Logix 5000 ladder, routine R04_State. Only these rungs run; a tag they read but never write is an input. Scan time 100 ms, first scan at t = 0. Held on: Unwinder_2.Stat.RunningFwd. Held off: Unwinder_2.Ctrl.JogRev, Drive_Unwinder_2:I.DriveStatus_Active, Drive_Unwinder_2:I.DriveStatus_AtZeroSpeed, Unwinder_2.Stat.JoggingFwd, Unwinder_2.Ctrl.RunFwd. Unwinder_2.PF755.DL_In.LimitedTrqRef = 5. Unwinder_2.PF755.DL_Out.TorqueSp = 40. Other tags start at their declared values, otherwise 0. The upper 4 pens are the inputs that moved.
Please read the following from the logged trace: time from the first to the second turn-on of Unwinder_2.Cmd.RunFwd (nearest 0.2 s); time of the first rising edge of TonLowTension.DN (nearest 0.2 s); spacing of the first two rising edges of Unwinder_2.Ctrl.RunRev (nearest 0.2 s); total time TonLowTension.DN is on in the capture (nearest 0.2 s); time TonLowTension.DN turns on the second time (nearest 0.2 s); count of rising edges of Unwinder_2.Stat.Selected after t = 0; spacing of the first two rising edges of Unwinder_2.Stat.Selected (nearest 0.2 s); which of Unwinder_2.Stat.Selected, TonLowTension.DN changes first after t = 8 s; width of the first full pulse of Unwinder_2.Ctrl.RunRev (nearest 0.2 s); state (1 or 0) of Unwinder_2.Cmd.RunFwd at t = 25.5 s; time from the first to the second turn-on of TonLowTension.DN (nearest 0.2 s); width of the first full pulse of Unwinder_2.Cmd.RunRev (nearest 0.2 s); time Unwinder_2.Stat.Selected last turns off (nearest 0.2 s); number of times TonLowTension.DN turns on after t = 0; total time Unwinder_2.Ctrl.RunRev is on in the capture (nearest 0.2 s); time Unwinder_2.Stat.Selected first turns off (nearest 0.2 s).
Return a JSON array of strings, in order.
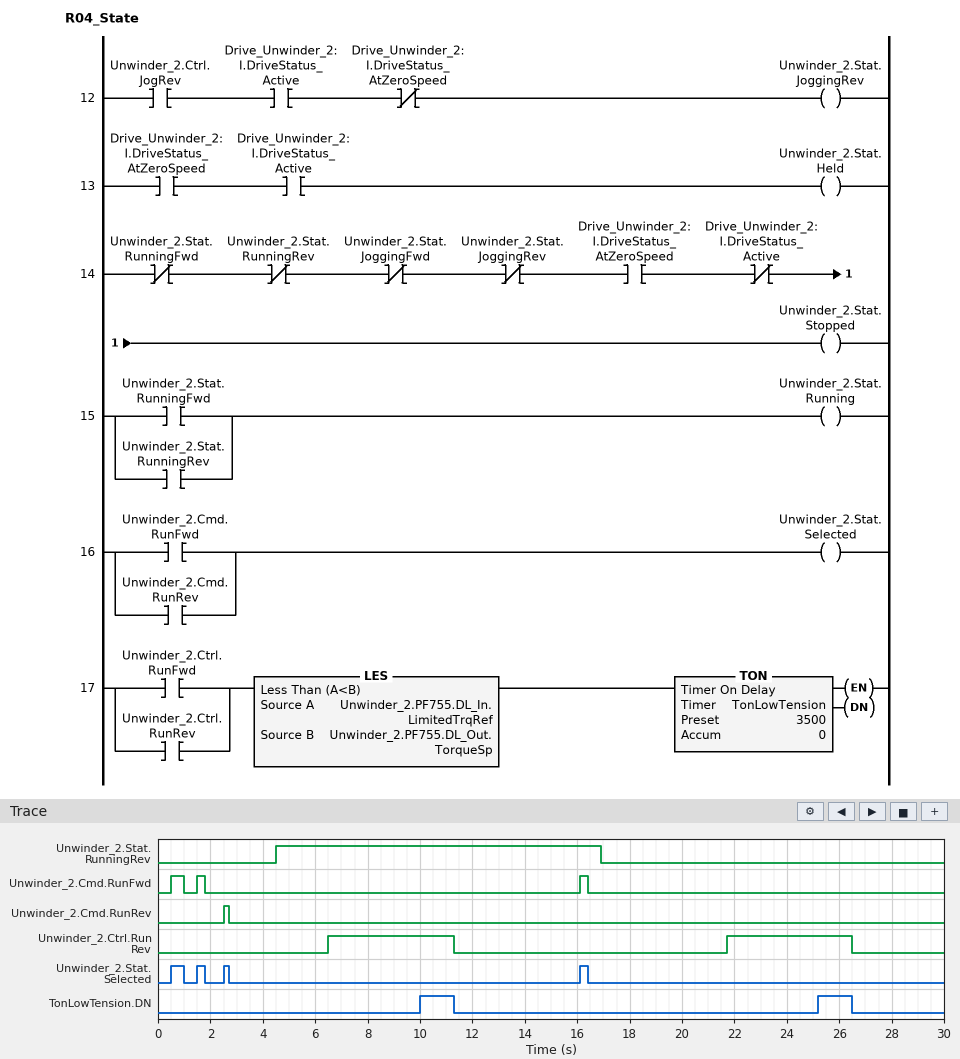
["1.0 s", "10.0 s", "15.2 s", "2.6 s", "25.2 s", "4", "1.0 s", "TonLowTension.DN", "4.8 s", "0", "15.2 s", "0.2 s", "16.4 s", "2", "9.6 s", "1.0 s"]
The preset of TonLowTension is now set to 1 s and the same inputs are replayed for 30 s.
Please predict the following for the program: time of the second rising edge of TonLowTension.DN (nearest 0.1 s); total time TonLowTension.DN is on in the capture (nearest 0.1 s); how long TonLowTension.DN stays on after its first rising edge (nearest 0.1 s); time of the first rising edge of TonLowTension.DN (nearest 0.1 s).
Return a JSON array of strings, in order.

["22.7 s", "7.6 s", "3.8 s", "7.5 s"]
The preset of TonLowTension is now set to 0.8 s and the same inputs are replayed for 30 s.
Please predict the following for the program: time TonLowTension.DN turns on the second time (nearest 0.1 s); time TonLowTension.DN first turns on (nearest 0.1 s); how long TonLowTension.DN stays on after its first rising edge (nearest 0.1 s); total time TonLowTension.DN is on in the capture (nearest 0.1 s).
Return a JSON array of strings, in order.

["22.5 s", "7.3 s", "4.0 s", "8.0 s"]
